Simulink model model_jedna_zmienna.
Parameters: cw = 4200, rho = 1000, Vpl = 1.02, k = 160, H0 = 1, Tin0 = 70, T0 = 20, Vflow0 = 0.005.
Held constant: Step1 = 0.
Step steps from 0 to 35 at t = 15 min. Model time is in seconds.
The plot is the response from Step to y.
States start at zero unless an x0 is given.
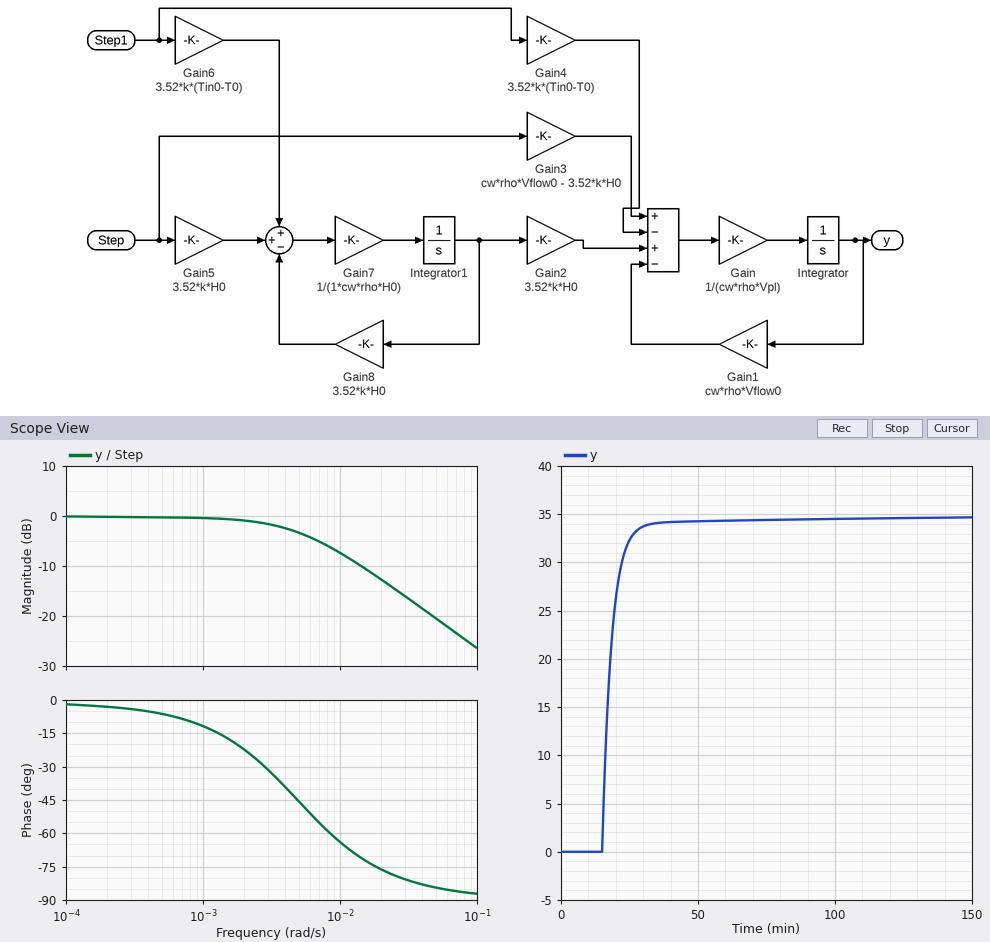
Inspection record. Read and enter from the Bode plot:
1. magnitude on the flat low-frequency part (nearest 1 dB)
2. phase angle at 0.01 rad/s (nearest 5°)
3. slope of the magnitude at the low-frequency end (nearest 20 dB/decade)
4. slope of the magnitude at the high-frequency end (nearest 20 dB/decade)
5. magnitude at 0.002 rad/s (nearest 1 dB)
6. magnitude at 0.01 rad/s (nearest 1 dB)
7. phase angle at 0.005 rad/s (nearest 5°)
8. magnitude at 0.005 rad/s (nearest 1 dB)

0 dB
-65°
0 dB/decade
-20 dB/decade
-1 dB
-7 dB
-45°
-3 dB
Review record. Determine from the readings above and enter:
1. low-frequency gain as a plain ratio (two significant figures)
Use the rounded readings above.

1.0
